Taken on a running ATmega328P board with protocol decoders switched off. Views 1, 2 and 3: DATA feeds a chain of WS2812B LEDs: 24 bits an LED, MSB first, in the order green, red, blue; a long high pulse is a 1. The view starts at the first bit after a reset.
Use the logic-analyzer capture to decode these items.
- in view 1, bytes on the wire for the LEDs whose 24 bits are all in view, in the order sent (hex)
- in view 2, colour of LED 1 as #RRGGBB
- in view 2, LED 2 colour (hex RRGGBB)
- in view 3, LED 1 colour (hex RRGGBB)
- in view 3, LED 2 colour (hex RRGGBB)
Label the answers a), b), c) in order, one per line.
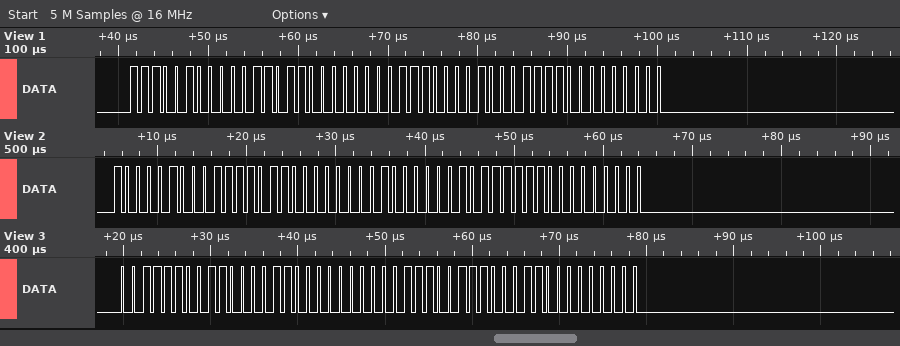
a) E4 1B 00 E1 1E 00
b) #7B8400
c) #7E8100
d) #C33C00
e) #C63900
